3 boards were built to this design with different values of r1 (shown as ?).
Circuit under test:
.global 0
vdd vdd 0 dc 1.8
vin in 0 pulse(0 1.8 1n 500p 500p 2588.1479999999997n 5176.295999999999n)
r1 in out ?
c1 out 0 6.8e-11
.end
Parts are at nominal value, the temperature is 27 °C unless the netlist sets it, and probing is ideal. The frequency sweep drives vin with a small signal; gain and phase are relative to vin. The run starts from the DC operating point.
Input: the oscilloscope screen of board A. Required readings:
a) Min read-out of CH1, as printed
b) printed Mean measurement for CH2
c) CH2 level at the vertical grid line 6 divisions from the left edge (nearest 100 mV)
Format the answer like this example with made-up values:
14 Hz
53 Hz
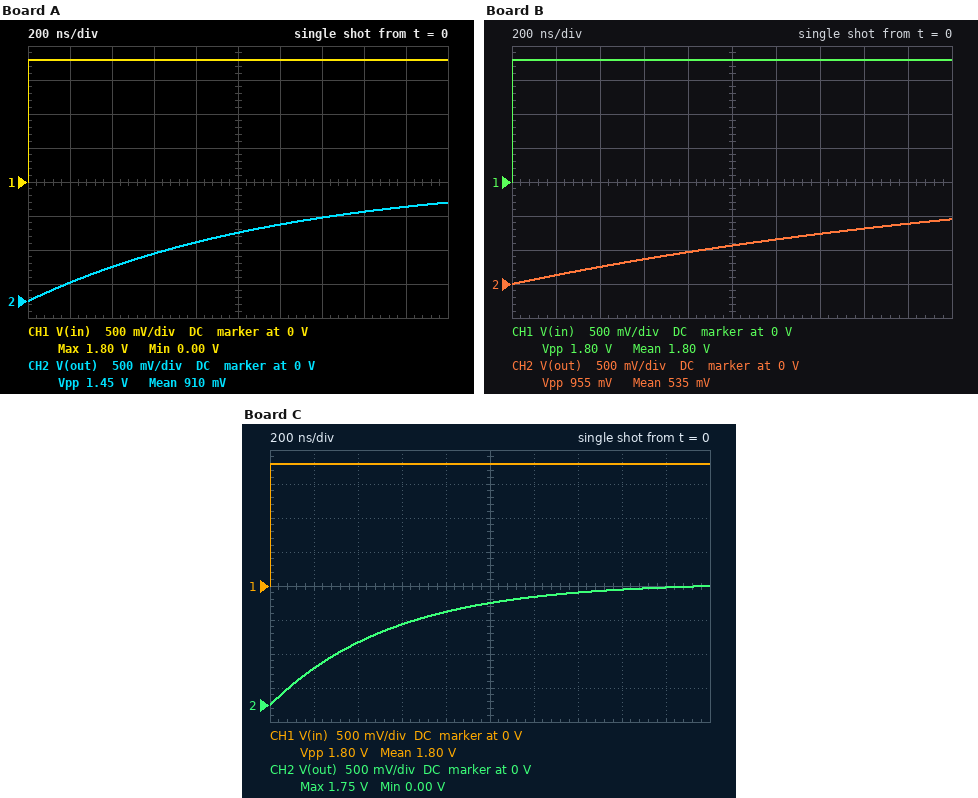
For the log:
0.00 V
910 mV
1.1 V
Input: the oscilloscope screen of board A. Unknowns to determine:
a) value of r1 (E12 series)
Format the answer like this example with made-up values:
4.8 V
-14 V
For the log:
18 kΩ
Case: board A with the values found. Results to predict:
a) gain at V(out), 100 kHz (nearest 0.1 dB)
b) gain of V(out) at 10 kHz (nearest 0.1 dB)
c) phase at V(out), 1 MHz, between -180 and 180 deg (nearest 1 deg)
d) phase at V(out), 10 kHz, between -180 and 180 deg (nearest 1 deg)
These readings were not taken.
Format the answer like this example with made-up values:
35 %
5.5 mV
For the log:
-2.0 dB
0 dB
-83 deg
-4 deg
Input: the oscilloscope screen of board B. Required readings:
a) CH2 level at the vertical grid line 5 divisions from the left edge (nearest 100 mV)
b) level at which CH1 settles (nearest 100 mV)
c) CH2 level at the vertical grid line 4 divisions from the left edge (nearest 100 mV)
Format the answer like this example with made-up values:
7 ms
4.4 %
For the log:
600 mV
1.8 V
500 mV
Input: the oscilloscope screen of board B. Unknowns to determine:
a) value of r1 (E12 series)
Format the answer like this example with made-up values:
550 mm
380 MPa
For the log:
39 kΩ
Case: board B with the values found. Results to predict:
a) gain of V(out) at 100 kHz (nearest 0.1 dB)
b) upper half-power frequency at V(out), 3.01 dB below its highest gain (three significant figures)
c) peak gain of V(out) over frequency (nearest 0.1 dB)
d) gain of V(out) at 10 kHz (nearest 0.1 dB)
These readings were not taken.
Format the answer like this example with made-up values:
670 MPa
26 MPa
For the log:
-5.8 dB
60.0 kHz
0 dB
-0.1 dB
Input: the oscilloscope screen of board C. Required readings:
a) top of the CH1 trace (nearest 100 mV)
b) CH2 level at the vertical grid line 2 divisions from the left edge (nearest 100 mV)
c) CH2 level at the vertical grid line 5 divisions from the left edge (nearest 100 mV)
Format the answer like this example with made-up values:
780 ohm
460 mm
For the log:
1.8 V
900 mV
1.5 V
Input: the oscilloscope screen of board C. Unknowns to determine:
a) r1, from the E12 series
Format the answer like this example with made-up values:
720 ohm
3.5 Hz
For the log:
8.2 kΩ
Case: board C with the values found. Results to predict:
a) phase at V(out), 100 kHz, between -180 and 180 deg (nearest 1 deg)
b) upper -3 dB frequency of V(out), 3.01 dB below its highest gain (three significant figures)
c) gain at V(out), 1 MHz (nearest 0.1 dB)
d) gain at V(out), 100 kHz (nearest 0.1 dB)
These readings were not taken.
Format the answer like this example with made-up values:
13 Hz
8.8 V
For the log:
-19 deg
285 kHz
-11.2 dB
-0.5 dB
